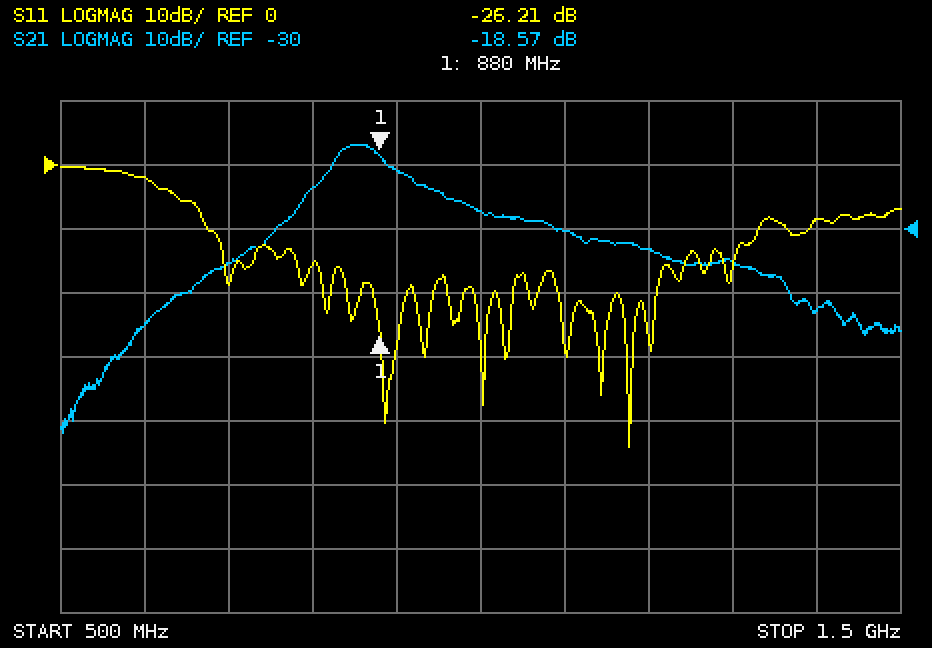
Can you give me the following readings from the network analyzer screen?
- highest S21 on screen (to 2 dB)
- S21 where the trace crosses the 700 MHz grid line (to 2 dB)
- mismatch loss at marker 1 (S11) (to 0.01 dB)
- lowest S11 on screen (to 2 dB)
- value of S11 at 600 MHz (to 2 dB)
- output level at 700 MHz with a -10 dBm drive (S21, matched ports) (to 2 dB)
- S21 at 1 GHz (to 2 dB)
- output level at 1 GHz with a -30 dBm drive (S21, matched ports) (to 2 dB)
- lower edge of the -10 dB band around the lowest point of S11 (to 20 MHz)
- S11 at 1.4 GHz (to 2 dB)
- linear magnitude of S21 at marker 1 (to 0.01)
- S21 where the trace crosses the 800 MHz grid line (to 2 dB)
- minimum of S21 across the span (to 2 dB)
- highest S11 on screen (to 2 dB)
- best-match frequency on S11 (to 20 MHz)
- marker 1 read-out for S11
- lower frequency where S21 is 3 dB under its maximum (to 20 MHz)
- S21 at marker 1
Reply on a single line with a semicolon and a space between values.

-16 dB; -36 dB; 0.01 dB; -44 dB; -2 dB; -46 dBm; -28 dB; -58 dBm; 680 MHz; -8 dB; 0.12; -24 dB; -62 dB; 0 dB; 1.18 GHz; -26.21 dB; 820 MHz; -18.57 dB
